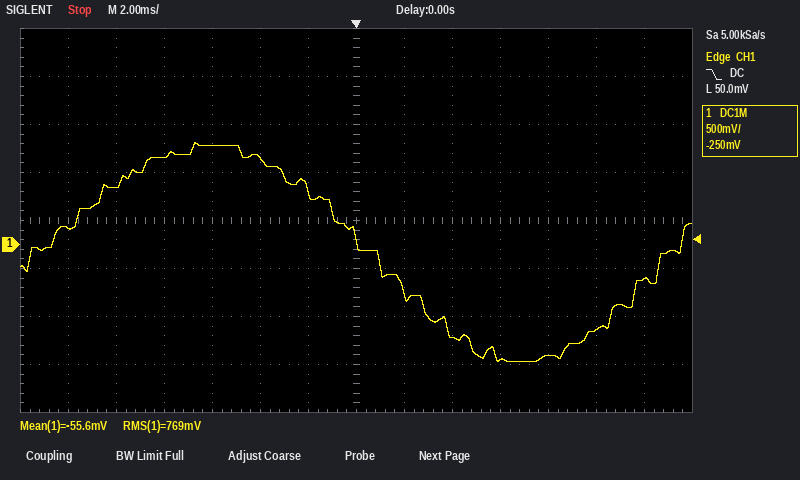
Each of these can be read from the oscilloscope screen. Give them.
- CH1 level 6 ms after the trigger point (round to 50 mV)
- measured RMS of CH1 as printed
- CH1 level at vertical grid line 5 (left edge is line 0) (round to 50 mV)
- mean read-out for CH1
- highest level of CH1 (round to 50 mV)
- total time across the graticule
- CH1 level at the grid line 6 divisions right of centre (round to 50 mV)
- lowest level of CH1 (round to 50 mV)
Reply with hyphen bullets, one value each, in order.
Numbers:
- -1.20 V
- 769 mV
- 900 mV
- -55.6 mV
- 1.05 V
- 28 ms
- -350 mV
- -1.20 V
